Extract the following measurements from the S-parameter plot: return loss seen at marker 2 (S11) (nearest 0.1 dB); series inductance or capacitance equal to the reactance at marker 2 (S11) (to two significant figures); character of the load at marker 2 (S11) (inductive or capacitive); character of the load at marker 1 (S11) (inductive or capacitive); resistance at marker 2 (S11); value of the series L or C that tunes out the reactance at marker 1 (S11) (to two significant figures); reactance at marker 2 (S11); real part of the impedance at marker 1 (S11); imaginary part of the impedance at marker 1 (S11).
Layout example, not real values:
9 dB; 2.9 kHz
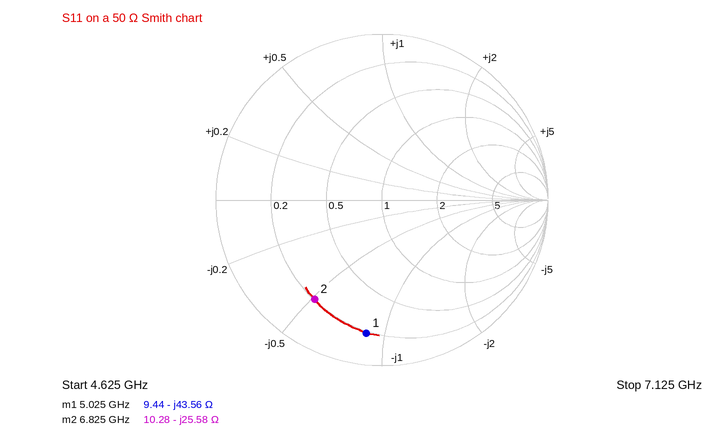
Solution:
2.8 dB; 910 fF; capacitive; capacitive; 10.28 Ω; 1.4 nH; -25.58 Ω; 9.44 Ω; -43.56 Ω
